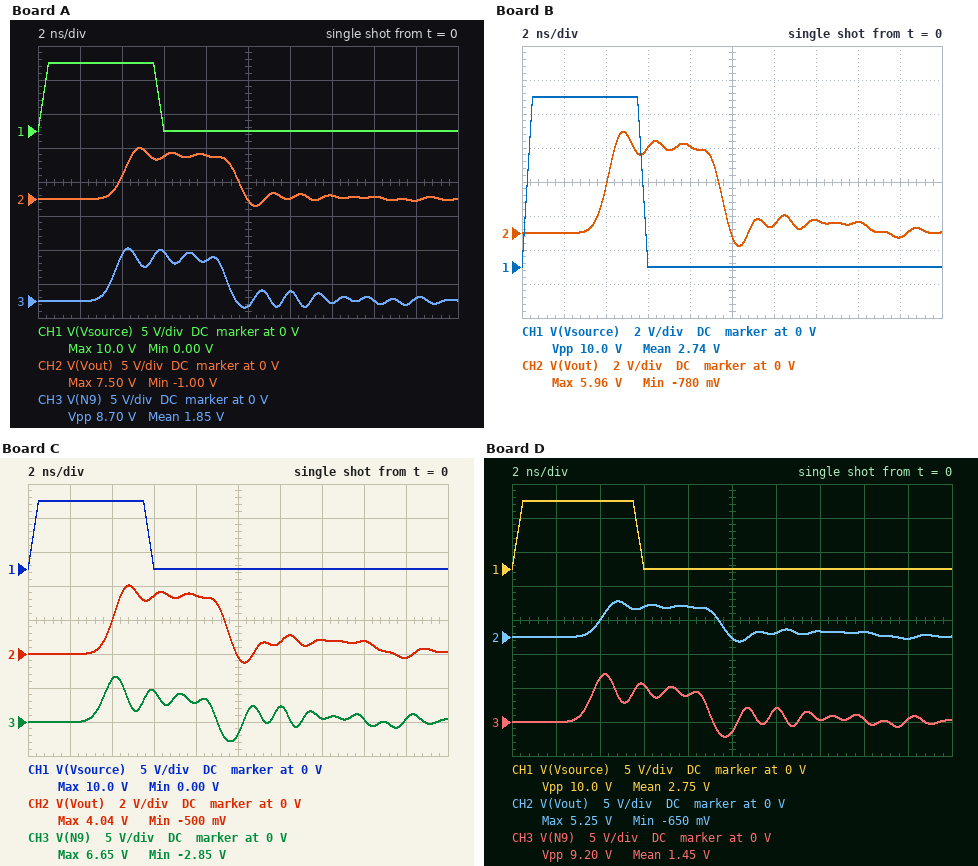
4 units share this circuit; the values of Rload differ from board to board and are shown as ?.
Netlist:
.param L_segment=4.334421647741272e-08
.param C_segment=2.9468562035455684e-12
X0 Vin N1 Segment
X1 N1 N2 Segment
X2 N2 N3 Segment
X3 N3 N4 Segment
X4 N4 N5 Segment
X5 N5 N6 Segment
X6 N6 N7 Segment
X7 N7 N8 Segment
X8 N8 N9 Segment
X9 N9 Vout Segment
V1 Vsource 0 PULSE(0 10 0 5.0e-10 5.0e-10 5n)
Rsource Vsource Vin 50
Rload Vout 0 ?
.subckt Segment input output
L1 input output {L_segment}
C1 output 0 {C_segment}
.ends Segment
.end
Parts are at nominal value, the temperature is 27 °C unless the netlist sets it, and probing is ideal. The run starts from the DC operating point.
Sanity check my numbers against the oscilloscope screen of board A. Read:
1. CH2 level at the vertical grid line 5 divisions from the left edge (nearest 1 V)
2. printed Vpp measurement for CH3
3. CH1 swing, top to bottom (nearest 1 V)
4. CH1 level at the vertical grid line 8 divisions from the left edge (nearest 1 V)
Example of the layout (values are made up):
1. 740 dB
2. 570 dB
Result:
1. 0 V
2. 8.70 V
3. 10 V
4. 0 V
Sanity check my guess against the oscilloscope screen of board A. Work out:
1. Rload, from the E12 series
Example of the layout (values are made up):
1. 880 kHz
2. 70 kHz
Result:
1. 100 Ω
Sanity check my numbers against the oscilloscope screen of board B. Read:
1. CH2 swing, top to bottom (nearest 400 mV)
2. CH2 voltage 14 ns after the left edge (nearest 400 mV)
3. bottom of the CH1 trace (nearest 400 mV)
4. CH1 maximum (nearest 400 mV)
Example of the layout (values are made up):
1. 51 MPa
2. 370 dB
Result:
1. 6.8 V
2. 800 mV
3. 0 V
4. 10.0 V
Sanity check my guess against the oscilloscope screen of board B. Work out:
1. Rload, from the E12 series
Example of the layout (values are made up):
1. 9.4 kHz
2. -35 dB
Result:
1. 68 Ω
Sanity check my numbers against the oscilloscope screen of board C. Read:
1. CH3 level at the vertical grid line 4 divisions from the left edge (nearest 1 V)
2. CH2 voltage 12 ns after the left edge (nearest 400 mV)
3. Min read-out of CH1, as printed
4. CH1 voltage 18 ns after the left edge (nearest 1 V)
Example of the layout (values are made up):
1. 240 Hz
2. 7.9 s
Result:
1. 3 V
2. 800 mV
3. 0.00 V
4. 0 V
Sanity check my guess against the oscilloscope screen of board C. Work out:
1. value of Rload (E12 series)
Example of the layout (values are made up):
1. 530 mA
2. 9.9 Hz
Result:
1. 39 Ω
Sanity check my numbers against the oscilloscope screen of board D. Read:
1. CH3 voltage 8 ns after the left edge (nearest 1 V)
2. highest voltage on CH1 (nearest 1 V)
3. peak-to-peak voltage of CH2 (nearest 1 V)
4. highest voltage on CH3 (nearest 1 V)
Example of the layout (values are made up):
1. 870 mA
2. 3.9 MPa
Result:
1. 4 V
2. 10 V
3. 6 V
4. 7 V
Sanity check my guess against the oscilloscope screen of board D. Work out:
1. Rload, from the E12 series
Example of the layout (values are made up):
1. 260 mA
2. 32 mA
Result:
1. 56 Ω
